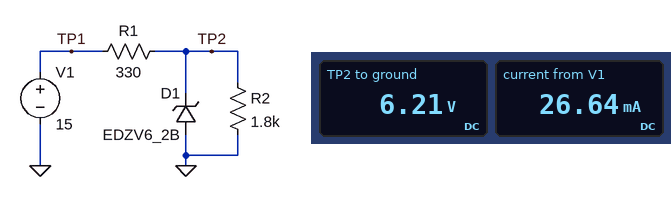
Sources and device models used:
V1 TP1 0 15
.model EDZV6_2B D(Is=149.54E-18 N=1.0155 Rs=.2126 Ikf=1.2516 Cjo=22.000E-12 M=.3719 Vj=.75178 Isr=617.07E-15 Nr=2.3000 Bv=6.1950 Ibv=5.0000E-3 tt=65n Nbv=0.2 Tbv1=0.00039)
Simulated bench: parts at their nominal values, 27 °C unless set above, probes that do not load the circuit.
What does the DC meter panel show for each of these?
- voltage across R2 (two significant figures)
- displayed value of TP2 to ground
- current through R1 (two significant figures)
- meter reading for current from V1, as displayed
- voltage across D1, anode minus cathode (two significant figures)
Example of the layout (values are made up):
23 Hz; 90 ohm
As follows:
6.2 V; 6.21 V; 27 mA; 26.64 mA; -6.2 V
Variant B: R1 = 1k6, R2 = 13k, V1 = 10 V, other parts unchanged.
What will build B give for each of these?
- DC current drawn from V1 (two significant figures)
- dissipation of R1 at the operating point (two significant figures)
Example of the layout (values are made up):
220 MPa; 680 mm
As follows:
2.4 mA; 9.1 mW
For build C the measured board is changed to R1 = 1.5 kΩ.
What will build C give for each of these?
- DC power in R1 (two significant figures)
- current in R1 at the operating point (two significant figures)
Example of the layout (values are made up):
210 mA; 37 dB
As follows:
52 mW; 5.9 mA
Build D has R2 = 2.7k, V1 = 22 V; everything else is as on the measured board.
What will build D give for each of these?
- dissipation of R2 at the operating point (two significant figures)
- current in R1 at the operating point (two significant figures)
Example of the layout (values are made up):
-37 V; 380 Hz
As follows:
14 mW; 48 mA
